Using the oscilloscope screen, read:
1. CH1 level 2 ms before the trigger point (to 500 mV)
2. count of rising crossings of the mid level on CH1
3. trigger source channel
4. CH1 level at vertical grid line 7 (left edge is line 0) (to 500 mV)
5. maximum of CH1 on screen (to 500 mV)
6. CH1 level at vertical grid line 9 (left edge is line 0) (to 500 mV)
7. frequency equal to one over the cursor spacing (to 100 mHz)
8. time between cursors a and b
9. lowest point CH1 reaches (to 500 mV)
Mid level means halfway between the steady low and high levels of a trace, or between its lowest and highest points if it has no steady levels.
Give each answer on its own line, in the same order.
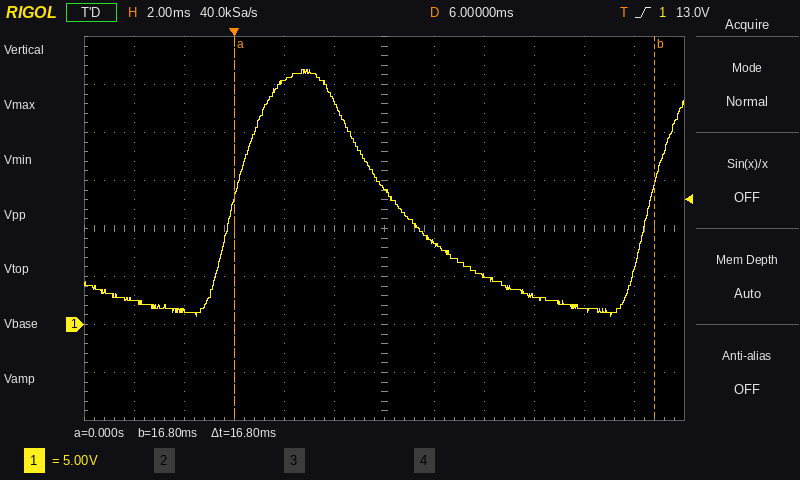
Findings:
1.5 V
2
CH1
8.5 V
26.5 V
3.0 V
59.5 Hz
16.8 ms
1.0 V
